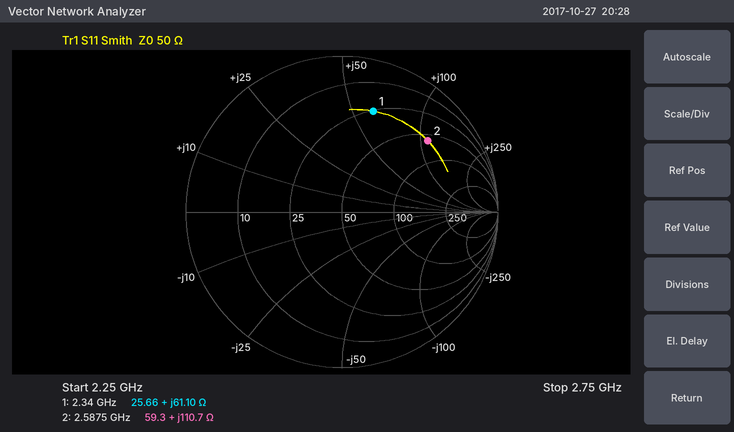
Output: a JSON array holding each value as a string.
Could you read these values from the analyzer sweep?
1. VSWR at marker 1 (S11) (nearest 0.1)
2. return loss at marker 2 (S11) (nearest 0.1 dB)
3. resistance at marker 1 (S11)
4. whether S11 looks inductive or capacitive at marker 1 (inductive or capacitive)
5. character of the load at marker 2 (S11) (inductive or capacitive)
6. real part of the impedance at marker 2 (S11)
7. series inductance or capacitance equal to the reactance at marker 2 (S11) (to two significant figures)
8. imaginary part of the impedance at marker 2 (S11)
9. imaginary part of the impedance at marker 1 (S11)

["5.2", "2.9 dB", "25.66 Ω", "inductive", "inductive", "59.3 Ω", "6.8 nH", "+110.7 Ω", "+61.10 Ω"]
